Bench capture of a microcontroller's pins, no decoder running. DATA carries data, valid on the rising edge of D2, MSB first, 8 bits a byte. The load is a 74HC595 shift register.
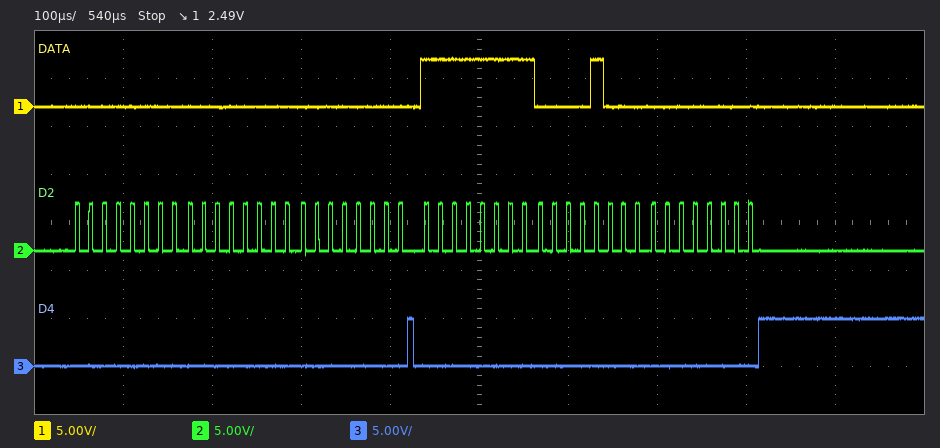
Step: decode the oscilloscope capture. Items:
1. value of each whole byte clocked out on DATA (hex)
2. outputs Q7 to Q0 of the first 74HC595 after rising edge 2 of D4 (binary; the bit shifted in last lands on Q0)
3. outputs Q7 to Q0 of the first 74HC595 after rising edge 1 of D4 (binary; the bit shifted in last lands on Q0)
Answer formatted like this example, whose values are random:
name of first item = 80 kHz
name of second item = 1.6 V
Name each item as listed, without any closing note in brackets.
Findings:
value of each whole byte clocked out on DATA = 00 00 00 FF 08 00
outputs Q7 to Q0 of the first 74HC595 after rising edge 2 of D4 = 00000000
outputs Q7 to Q0 of the first 74HC595 after rising edge 1 of D4 = 00000000
